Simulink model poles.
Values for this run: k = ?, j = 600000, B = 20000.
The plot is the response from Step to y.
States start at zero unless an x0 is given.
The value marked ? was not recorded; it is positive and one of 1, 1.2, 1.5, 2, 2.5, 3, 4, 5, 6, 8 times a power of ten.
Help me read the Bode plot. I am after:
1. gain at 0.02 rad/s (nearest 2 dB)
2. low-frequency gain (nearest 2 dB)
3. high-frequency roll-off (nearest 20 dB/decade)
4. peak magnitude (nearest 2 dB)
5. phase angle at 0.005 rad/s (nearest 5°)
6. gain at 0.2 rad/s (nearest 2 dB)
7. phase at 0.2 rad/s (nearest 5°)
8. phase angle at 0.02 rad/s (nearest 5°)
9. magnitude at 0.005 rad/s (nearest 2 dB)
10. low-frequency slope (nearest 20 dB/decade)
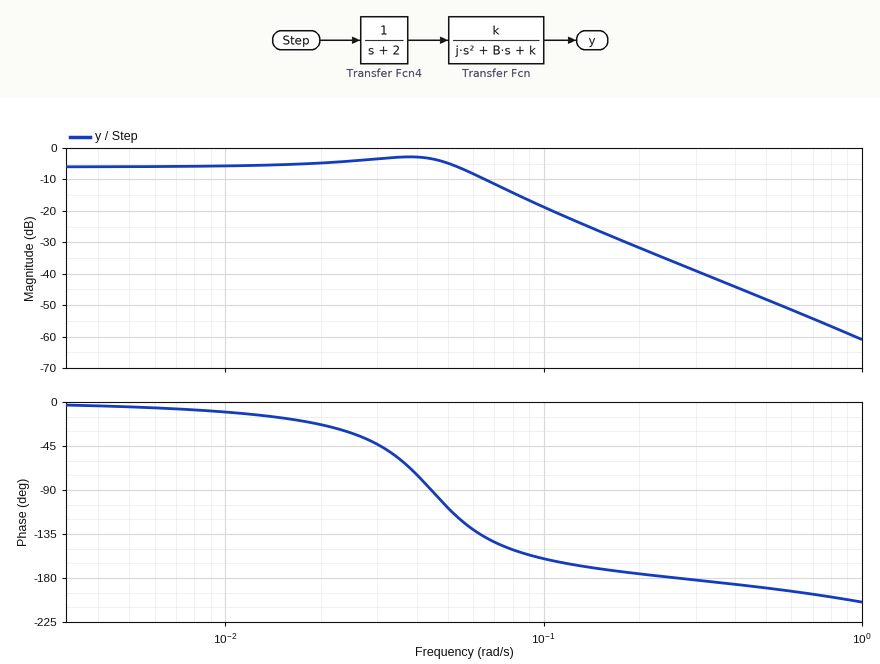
-4 dB
-6 dB
-40 dB/decade
-2 dB
-5°
-32 dB
-175°
-25°
-6 dB
0 dB/decade
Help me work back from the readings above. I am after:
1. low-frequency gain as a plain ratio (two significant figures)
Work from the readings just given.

0.50
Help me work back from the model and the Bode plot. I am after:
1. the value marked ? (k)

1200
